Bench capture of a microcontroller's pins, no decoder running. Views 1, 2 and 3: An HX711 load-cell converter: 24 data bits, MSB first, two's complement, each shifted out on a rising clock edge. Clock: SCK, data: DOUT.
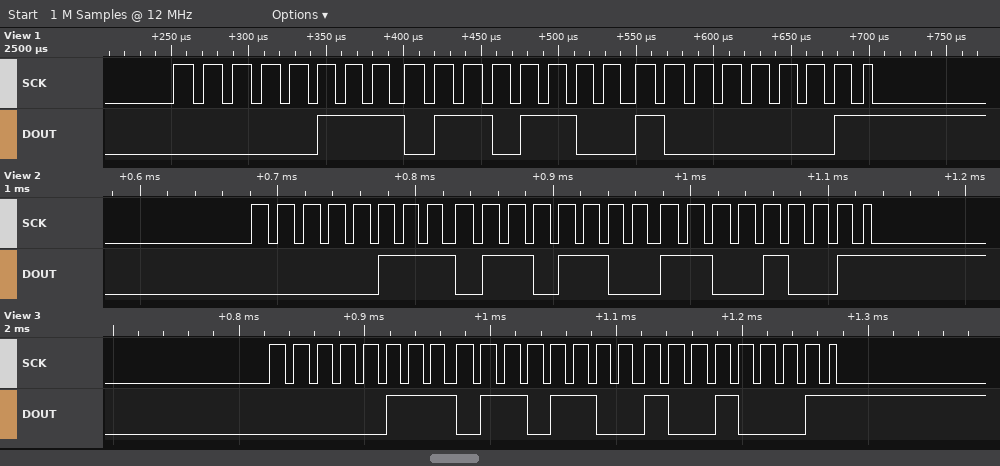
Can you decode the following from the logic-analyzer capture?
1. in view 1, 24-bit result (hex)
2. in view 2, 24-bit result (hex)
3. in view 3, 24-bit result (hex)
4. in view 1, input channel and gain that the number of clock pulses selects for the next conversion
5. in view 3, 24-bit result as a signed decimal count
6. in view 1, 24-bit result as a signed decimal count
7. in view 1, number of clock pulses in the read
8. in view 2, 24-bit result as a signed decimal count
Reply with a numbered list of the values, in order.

1. 0x076C81
2. 0x076CC9
3. 0x076C91
4. channel A, gain 128
5. 486545
6. 486529
7. 25
8. 486601
